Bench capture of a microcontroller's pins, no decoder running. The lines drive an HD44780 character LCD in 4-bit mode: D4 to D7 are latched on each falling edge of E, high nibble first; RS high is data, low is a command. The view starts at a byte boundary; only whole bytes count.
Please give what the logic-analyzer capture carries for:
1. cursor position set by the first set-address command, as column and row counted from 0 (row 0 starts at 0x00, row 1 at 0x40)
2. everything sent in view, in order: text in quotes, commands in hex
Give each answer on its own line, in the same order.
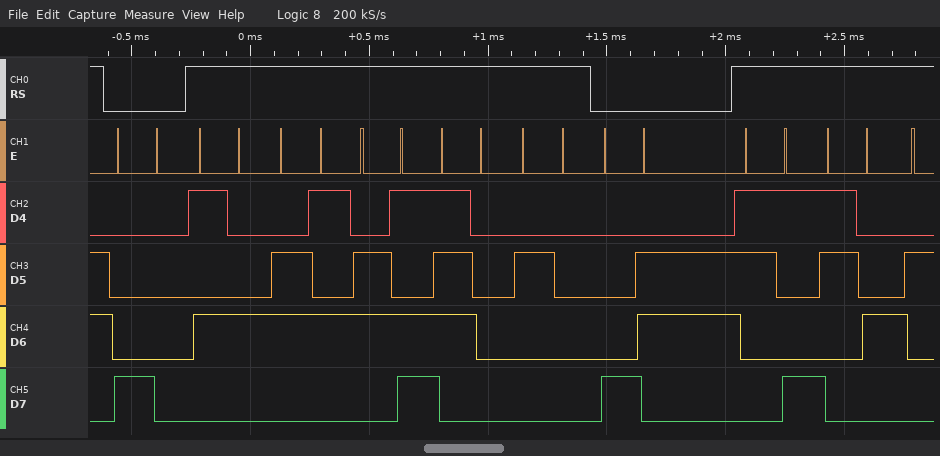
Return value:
column 0, row 0
0x80 "Temp " 0x86 "94"
